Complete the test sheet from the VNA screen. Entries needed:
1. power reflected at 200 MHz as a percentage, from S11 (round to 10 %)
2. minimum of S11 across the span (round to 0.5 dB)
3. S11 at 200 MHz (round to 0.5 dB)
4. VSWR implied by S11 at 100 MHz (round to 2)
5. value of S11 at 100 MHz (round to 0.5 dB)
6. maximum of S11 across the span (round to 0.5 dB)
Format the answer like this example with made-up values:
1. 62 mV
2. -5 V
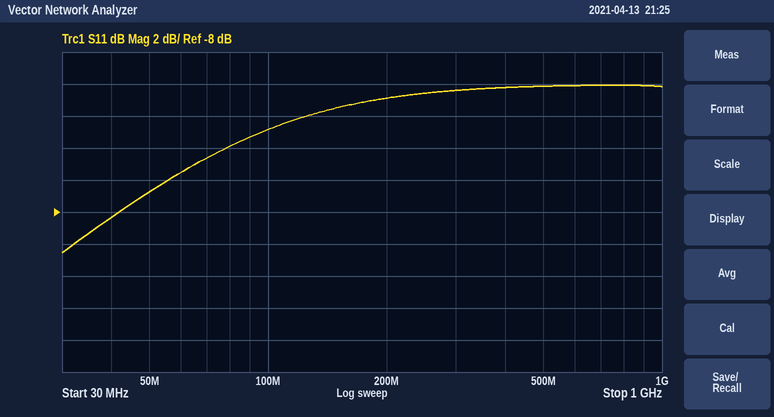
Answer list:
1. 80 %
2. -10.5 dB
3. -1.0 dB
4. 6
5. -3.0 dB
6. 0.0 dB
